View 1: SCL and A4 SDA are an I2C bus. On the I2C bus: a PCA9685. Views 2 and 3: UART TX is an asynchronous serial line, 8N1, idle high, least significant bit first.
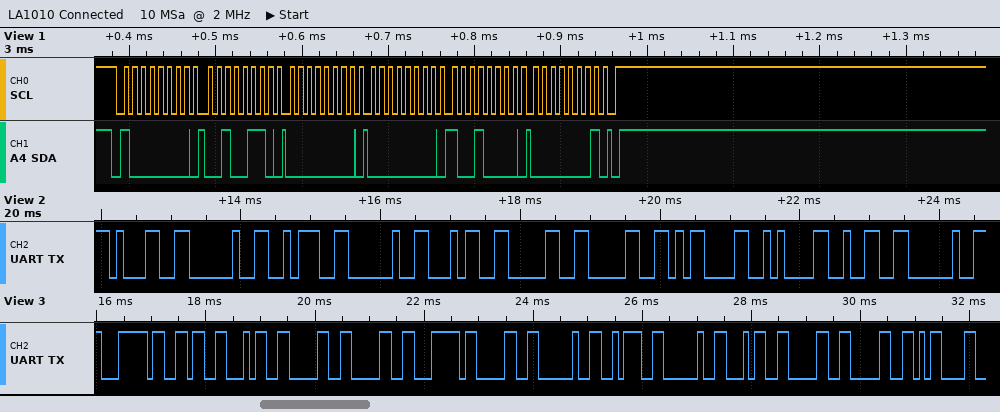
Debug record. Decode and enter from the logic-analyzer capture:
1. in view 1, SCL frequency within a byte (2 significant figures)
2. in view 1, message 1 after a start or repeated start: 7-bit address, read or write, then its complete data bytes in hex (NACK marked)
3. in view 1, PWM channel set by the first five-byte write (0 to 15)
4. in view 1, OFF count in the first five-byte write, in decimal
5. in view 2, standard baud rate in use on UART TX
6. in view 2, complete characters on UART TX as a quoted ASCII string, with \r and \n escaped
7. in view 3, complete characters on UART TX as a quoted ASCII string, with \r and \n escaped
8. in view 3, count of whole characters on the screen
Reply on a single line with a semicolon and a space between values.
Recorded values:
100 kHz; 0x40 write: 26 00 00 90 01; 8; 400; 9600 baud; "1 : 400\r\n2 "; "|6400|0 : 400\r"; 14
